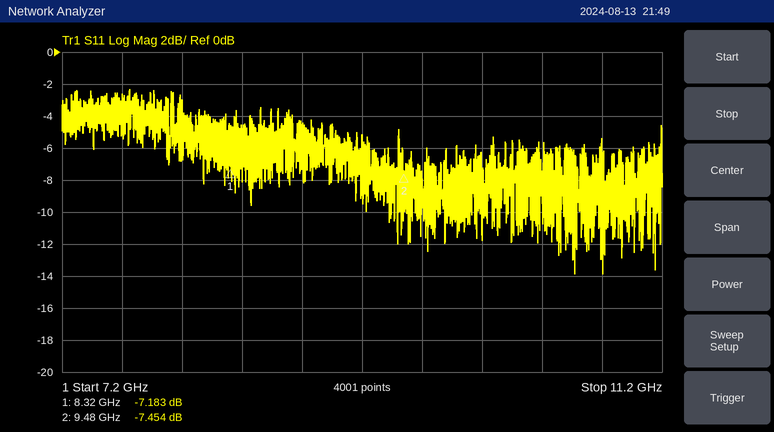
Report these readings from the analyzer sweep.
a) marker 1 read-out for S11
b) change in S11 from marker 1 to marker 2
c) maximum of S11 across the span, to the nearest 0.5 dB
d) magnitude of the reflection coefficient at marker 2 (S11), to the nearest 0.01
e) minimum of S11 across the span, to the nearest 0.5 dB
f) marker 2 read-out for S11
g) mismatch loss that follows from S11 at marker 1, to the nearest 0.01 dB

-7.183 dB
-0.271 dB
-2.5 dB
0.42
-14.0 dB
-7.454 dB
0.92 dB
